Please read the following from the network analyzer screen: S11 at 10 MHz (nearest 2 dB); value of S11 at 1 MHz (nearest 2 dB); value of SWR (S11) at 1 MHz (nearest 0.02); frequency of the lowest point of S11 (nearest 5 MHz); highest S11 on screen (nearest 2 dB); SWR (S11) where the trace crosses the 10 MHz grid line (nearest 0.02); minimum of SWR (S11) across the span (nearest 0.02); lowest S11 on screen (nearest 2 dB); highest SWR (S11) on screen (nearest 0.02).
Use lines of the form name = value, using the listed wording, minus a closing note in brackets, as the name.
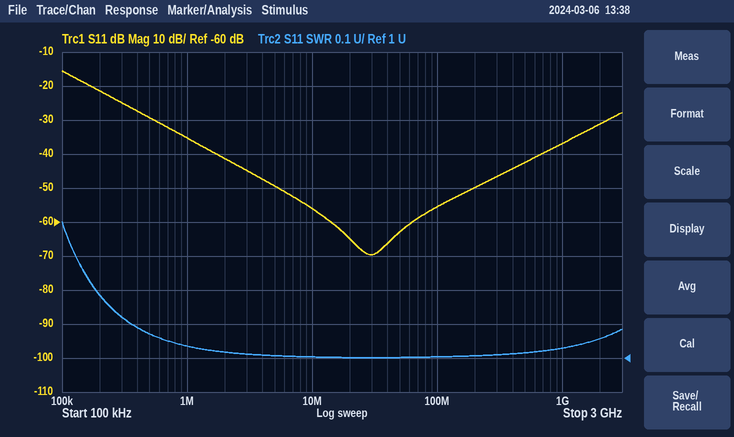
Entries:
S11 at 10 MHz = -56 dB
value of S11 at 1 MHz = -36 dB
value of SWR (S11) at 1 MHz = 1.04
frequency of the lowest point of S11 = 30 MHz
highest S11 on screen = -16 dB
SWR (S11) where the trace crosses the 10 MHz grid line = 1.00
minimum of SWR (S11) across the span = 1.00
lowest S11 on screen = -70 dB
highest SWR (S11) on screen = 1.40
